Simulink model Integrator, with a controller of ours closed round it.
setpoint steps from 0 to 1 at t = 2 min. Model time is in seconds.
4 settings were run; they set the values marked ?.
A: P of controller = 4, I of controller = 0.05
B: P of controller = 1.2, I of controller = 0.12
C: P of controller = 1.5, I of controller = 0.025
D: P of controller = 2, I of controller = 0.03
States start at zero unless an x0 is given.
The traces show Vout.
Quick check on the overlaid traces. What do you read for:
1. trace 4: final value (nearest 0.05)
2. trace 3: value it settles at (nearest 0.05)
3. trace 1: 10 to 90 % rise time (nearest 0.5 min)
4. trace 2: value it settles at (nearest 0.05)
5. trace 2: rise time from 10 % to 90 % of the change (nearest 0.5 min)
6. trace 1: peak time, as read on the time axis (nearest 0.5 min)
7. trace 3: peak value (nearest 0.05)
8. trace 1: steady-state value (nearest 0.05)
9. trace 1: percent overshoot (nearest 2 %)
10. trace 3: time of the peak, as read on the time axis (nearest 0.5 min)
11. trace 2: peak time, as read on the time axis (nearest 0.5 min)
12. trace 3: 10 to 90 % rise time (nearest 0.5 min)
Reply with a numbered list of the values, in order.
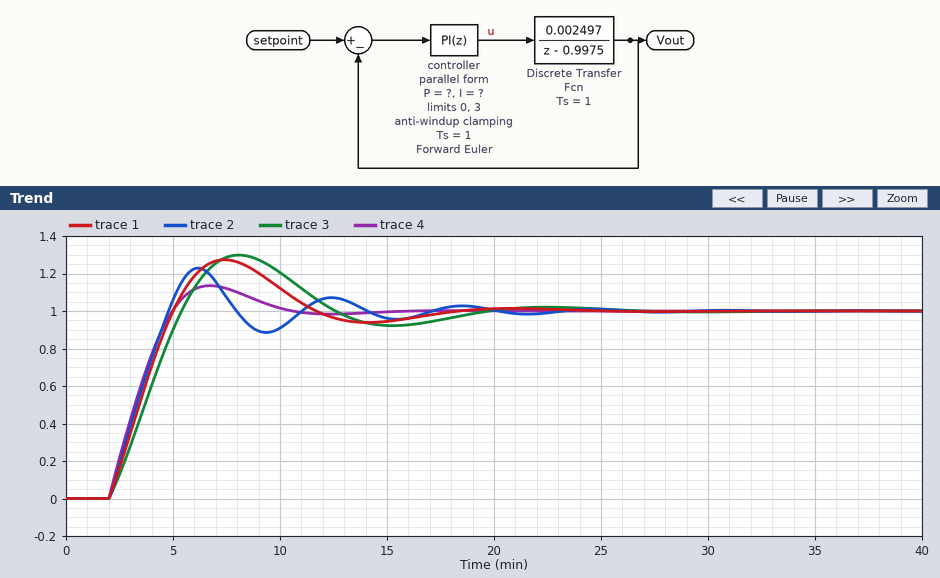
1. 1.00
2. 1.00
3. 2.5 min
4. 1.00
5. 2.0 min
6. 7.5 min
7. 1.30
8. 1.00
9. 28 %
10. 8.0 min
11. 6.0 min
12. 2.5 min
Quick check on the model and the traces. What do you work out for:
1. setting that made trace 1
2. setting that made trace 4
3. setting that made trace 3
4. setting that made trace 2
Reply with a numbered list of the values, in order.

1. D
2. A
3. C
4. B
